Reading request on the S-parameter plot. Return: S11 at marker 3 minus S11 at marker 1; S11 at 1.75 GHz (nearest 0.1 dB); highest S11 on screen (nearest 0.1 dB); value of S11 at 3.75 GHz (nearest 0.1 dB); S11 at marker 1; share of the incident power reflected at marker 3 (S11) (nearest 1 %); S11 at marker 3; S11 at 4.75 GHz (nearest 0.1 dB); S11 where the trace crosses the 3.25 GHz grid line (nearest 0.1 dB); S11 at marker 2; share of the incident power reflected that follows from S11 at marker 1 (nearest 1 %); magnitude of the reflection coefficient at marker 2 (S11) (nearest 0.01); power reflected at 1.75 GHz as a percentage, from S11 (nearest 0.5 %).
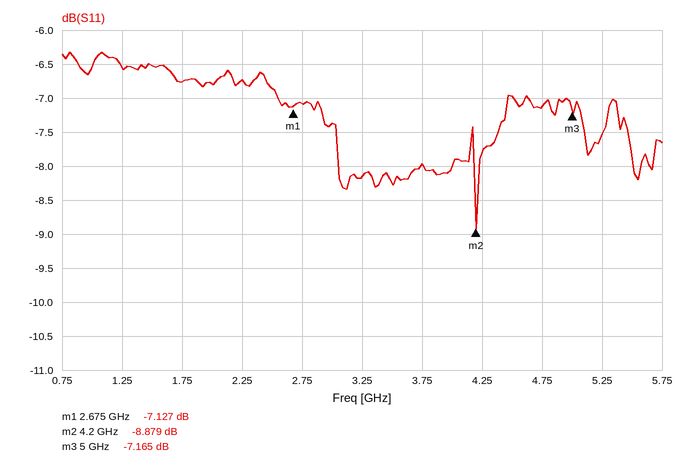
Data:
-0.038 dB
-6.8 dB
-6.3 dB
-8.0 dB
-7.127 dB
19 %
-7.165 dB
-7.1 dB
-8.2 dB
-8.879 dB
19 %
0.36
21.0 %
